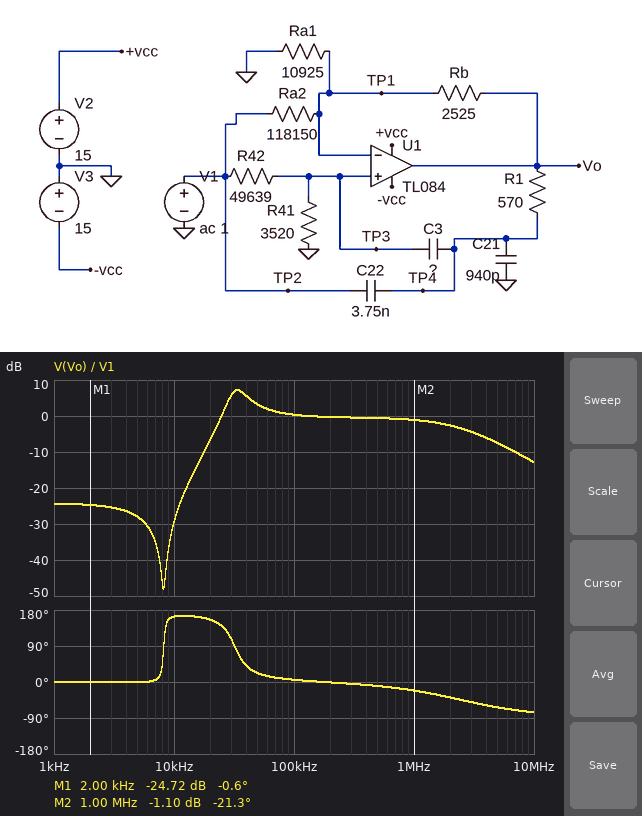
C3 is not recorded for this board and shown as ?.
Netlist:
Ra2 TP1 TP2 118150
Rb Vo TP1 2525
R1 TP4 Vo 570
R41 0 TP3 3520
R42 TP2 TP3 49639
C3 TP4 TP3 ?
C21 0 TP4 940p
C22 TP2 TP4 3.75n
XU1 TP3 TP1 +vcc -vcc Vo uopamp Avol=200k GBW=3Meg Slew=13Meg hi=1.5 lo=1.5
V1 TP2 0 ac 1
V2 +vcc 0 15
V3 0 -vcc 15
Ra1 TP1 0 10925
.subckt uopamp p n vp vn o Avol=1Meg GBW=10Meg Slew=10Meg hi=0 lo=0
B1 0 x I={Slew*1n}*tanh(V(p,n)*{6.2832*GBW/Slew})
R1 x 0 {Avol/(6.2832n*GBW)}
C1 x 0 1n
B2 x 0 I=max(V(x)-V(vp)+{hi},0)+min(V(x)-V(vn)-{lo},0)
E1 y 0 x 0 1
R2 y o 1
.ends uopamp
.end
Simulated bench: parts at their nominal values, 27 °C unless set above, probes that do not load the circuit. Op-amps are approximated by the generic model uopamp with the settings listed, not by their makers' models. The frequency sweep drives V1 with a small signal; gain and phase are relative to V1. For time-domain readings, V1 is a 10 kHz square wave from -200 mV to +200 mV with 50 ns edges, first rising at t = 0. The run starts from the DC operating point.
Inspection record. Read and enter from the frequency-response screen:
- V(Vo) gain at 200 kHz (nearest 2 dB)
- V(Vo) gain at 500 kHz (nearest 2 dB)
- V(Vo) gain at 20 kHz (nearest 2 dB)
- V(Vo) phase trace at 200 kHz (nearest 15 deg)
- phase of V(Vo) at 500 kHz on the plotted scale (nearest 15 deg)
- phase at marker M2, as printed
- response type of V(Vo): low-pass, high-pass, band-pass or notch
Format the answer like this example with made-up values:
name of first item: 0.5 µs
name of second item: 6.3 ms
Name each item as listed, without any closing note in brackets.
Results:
V(Vo) gain at 200 kHz: 0 dB
V(Vo) gain at 500 kHz: 0 dB
V(Vo) gain at 20 kHz: -6 dB
V(Vo) phase trace at 200 kHz: 0 deg
phase of V(Vo) at 500 kHz on the plotted scale: -15 deg
phase at marker M2, as printed: -21.3 deg
response type of V(Vo): low-pass, high-pass, band-pass or notch: band-pass
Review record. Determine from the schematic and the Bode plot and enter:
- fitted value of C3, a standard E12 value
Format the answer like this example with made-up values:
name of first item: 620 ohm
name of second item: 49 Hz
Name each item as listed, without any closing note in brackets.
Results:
fitted value of C3, a standard E12 value: 2.7 nF
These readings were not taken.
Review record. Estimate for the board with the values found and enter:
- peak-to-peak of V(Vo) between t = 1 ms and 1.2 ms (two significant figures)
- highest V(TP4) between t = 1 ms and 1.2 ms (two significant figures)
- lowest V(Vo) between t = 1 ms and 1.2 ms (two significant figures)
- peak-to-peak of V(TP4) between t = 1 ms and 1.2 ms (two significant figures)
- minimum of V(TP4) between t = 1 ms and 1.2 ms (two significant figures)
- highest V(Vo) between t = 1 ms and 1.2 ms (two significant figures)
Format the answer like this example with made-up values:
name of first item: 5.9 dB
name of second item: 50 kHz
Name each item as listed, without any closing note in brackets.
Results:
peak-to-peak of V(Vo) between t = 1 ms and 1.2 ms: 790 mV
highest V(TP4) between t = 1 ms and 1.2 ms: 350 mV
lowest V(Vo) between t = 1 ms and 1.2 ms: -400 mV
peak-to-peak of V(TP4) between t = 1 ms and 1.2 ms: 700 mV
minimum of V(TP4) between t = 1 ms and 1.2 ms: -350 mV
highest V(Vo) between t = 1 ms and 1.2 ms: 400 mV
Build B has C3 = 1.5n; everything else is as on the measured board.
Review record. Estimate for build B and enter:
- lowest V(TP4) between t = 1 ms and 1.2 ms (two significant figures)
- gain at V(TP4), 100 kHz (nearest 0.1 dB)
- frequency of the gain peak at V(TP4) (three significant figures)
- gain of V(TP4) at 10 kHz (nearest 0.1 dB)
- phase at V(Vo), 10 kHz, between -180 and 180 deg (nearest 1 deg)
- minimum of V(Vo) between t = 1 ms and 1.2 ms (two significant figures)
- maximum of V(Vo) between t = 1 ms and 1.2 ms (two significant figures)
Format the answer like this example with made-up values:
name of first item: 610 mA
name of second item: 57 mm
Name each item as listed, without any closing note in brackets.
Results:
lowest V(TP4) between t = 1 ms and 1.2 ms: -300 mV
gain at V(TP4), 100 kHz: -0.6 dB
frequency of the gain peak at V(TP4): 46.6 kHz
gain of V(TP4) at 10 kHz: -17.2 dB
phase at V(Vo), 10 kHz, between -180 and 180 deg: 25 deg
minimum of V(Vo) between t = 1 ms and 1.2 ms: -350 mV
maximum of V(Vo) between t = 1 ms and 1.2 ms: 350 mV
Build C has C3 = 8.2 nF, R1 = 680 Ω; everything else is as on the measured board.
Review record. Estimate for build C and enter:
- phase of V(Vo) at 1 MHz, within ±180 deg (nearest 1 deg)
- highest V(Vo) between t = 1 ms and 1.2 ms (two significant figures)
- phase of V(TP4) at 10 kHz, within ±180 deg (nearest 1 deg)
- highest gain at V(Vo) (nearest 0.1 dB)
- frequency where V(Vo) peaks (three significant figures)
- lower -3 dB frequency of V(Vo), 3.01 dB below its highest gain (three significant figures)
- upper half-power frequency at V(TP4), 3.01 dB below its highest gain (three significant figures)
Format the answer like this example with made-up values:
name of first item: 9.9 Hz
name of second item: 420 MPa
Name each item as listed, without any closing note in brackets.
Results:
phase of V(Vo) at 1 MHz, within ±180 deg: -22 deg
highest V(Vo) between t = 1 ms and 1.2 ms: 240 mV
phase of V(TP4) at 10 kHz, within ±180 deg: 134 deg
highest gain at V(Vo): 12.7 dB
frequency where V(Vo) peaks: 17.2 kHz
lower -3 dB frequency of V(Vo), 3.01 dB below its highest gain: 15.6 kHz
upper half-power frequency at V(TP4), 3.01 dB below its highest gain: 19.3 kHz
